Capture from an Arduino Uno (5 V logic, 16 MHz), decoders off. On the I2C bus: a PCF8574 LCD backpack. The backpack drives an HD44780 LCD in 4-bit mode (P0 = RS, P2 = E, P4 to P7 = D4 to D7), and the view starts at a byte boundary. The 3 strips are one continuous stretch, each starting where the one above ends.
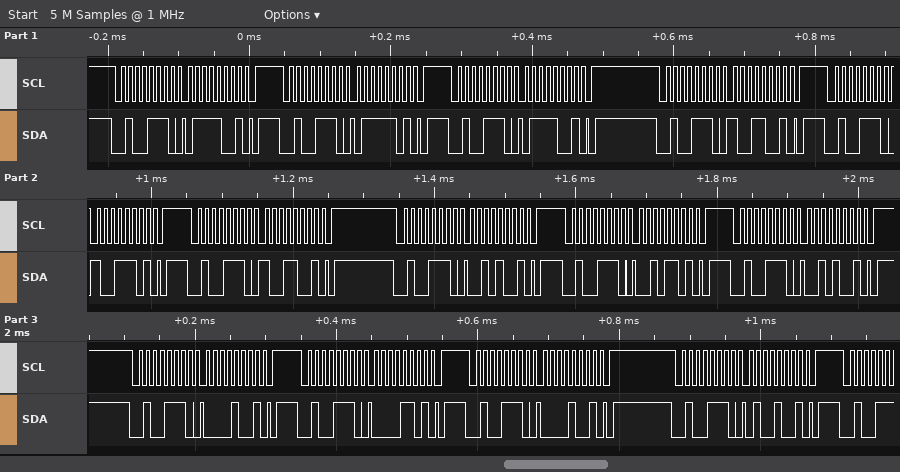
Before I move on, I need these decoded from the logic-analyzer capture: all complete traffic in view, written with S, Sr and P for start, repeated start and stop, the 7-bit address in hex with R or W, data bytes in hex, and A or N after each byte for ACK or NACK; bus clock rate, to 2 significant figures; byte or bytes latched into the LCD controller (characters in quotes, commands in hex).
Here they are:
S 27W A 79 A P S 27W A 7D A P S 27W A 79 A P S 27W A 99 A P S 27W A 9D A P S 27W A 99 A P S 27W A 29 A P S 27W A 2D A P S 27W A 29 A P S 27W A 09 A P S 27W A 0D A P S 27W A 09 A P S 27W A 49 A P
100 kHz
'y' ' '
